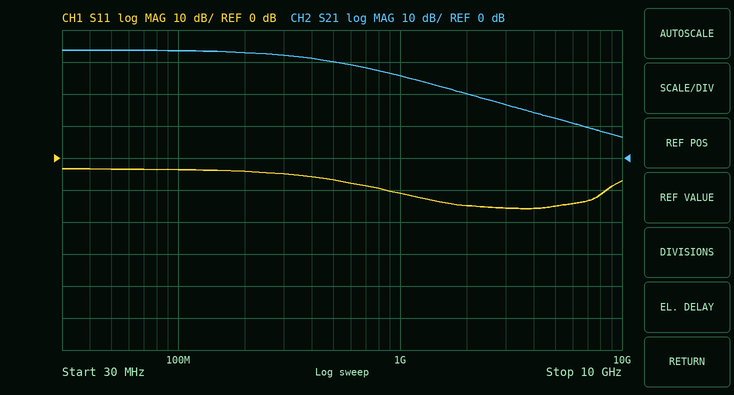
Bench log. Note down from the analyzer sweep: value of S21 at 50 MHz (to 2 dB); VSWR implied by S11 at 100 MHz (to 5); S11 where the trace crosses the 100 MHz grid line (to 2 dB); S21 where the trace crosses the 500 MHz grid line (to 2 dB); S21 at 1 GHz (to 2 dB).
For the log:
34 dB
5
-4 dB
30 dB
26 dB
